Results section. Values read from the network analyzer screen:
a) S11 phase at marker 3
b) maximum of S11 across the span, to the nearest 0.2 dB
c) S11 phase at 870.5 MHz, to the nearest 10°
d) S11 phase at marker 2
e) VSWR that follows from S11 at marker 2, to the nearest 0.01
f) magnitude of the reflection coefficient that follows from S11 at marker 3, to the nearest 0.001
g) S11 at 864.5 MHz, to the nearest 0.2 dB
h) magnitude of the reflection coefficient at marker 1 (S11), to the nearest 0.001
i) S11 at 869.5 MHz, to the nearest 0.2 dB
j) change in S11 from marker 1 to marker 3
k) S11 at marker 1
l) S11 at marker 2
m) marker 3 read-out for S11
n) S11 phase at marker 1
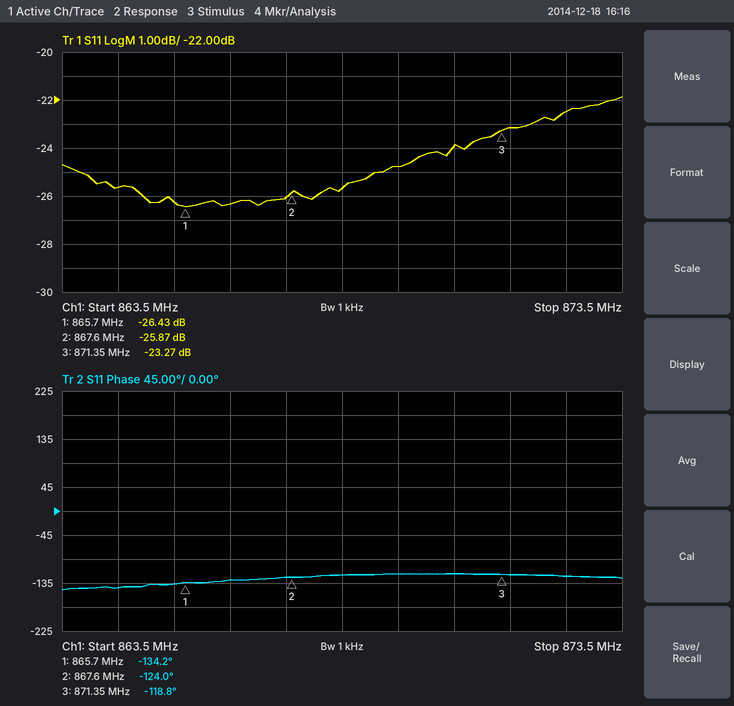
-118.8°
-21.8 dB
-120°
-124.0°
1.11
0.069
-25.6 dB
0.048
-24.8 dB
3.16 dB
-26.43 dB
-25.87 dB
-23.27 dB
-134.2°
